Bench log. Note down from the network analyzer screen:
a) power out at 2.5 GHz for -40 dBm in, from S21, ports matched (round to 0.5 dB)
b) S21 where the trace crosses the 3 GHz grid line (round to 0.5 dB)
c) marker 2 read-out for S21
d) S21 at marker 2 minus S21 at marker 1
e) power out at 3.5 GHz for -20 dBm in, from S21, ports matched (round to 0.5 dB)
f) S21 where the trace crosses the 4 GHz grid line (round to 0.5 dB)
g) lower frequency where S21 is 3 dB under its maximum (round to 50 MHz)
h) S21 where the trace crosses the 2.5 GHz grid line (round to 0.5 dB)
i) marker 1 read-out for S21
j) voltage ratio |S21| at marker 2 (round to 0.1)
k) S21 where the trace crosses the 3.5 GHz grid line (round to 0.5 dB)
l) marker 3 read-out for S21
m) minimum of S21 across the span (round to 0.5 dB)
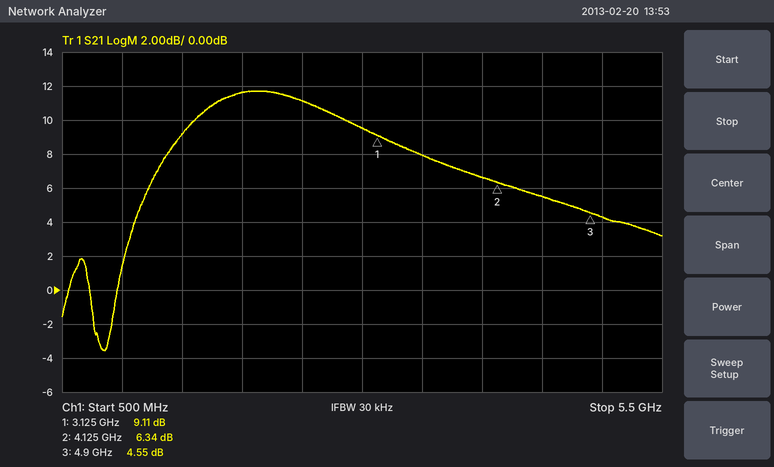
-29.0 dBm
9.5 dB
6.34 dB
-2.77 dB
-12.0 dBm
6.5 dB
1.45 GHz
11.0 dB
9.11 dB
2.1
8.0 dB
4.55 dB
-3.5 dB
